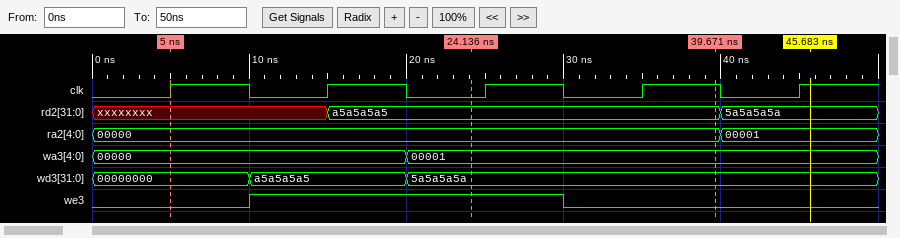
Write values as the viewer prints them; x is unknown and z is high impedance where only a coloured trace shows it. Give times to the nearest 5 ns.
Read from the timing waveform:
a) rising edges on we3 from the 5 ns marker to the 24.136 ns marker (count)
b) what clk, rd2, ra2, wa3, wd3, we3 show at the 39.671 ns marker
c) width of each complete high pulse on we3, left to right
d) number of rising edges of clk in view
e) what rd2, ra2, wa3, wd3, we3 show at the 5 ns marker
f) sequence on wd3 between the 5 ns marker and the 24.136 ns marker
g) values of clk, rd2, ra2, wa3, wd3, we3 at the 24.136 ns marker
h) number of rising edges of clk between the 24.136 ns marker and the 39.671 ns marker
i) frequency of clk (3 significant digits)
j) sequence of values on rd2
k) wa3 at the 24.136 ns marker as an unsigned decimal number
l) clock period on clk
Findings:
1
clk=1, rd2=a5a5a5a5, ra2=00000, wa3=00001, wd3=5a5a5a5a, we3=0
20 ns
5
rd2=xxxxxxxx, ra2=00000, wa3=00000, wd3=00000000, we3=0
00000000, a5a5a5a5, 5a5a5a5a
clk=0, rd2=a5a5a5a5, ra2=00000, wa3=00001, wd3=5a5a5a5a, we3=1
2
100 MHz
xxxxxxxx, a5a5a5a5, 5a5a5a5a
1
10 ns
